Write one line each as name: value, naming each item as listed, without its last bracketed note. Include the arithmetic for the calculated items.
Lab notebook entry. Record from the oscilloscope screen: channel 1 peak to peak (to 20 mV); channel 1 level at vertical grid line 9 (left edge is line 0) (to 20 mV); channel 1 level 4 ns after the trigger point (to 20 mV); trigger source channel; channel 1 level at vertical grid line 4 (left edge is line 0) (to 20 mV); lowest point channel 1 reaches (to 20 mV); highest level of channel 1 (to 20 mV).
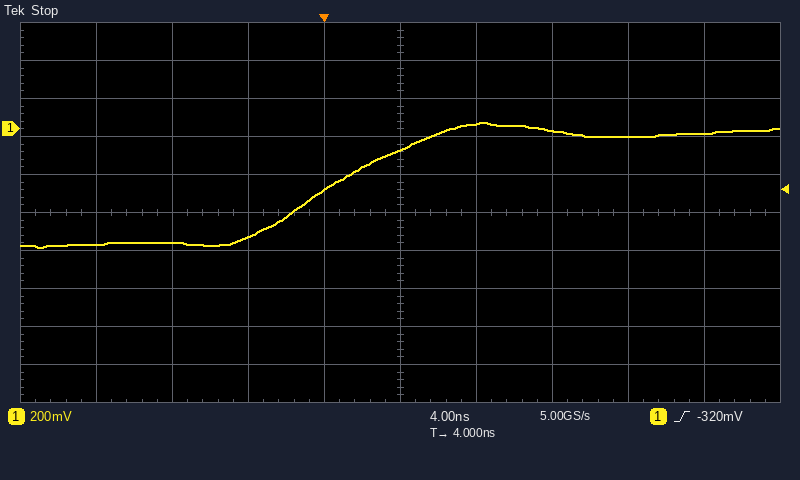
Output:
channel 1 peak to peak: 40 mV − (-620 mV) = 660 mV
channel 1 level at vertical grid line 9 (left edge is line 0): -20 mV
channel 1 level 4 ns after the trigger point: -120 mV
trigger source channel: channel 1
channel 1 level at vertical grid line 4 (left edge is line 0): -320 mV
lowest point channel 1 reaches: -620 mV
highest level of channel 1: 40 mV
